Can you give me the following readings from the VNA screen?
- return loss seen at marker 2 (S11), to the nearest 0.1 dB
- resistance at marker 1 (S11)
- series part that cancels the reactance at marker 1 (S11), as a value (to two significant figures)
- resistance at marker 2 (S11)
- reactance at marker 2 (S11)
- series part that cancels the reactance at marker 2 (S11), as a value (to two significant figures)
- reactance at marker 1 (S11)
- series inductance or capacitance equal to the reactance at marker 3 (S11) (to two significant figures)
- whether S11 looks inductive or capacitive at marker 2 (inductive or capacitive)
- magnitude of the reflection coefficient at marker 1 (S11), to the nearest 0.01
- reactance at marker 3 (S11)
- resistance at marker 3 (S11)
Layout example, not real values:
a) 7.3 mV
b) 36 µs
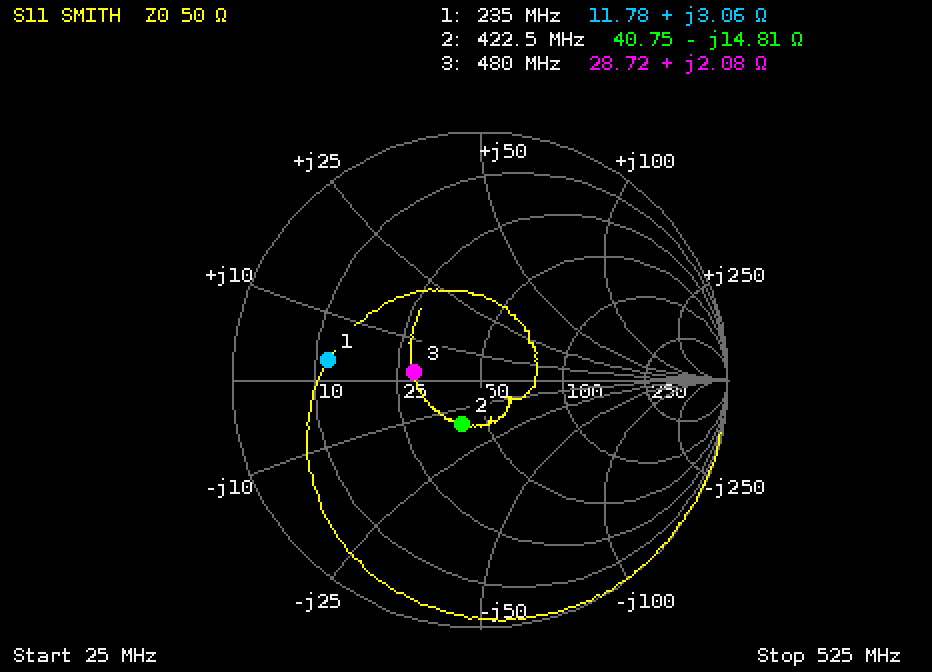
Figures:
a) 14.4 dB
b) 11.78 Ω
c) 220 pF
d) 40.75 Ω
e) -14.81 Ω
f) 5.6 nH
g) +3.06 Ω
h) 690 pH
i) capacitive
j) 0.62
k) +2.08 Ω
l) 28.72 Ω
